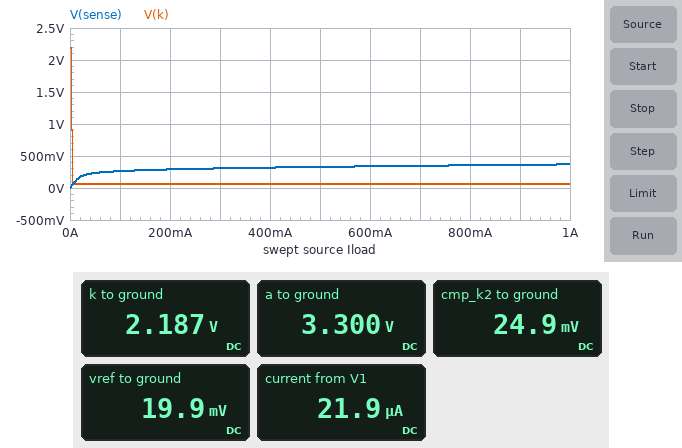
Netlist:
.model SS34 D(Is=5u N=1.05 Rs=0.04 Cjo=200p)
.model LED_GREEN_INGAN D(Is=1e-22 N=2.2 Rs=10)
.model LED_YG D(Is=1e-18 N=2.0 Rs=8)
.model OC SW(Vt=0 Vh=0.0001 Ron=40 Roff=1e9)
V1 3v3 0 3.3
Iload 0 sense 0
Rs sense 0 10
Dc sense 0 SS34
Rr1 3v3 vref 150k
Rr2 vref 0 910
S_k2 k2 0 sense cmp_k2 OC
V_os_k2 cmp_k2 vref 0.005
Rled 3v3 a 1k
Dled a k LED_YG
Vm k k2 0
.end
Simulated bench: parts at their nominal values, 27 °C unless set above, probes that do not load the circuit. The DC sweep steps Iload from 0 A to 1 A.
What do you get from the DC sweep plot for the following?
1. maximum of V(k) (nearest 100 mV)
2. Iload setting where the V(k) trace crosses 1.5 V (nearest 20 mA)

2.2 V
0 A
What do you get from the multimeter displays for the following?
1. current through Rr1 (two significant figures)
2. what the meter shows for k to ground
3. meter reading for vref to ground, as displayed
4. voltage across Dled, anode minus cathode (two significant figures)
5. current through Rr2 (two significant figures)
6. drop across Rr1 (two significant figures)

22 µA
2.187 V
19.9 mV
1.1 V
22 µA
3.3 V
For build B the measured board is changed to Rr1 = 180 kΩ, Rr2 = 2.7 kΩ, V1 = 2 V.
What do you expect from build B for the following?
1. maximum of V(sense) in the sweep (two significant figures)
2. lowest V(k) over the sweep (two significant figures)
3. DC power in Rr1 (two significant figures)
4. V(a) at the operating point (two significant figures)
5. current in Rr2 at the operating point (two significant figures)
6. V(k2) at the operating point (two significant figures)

370 mV
11 mV
22 µW
2.0 V
11 µA
930 mV
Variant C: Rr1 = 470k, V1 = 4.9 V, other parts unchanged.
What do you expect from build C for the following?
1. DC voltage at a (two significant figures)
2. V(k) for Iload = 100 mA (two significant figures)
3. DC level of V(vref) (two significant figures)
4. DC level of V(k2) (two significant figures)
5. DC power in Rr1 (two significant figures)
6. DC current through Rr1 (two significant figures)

4.9 V
120 mV
9.5 mV
3.8 V
51 µW
10 µA
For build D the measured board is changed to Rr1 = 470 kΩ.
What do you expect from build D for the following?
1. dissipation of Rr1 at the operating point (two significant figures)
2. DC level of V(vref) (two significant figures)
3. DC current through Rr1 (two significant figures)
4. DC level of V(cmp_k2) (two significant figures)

23 µW
6.4 mV
7.0 µA
11 mV
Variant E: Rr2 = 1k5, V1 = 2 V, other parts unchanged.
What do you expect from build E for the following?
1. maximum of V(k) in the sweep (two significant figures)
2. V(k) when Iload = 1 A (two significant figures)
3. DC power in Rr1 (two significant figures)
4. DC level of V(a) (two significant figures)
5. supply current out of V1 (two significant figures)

930 mV
11 mV
26 µW
2.0 V
13 µA
